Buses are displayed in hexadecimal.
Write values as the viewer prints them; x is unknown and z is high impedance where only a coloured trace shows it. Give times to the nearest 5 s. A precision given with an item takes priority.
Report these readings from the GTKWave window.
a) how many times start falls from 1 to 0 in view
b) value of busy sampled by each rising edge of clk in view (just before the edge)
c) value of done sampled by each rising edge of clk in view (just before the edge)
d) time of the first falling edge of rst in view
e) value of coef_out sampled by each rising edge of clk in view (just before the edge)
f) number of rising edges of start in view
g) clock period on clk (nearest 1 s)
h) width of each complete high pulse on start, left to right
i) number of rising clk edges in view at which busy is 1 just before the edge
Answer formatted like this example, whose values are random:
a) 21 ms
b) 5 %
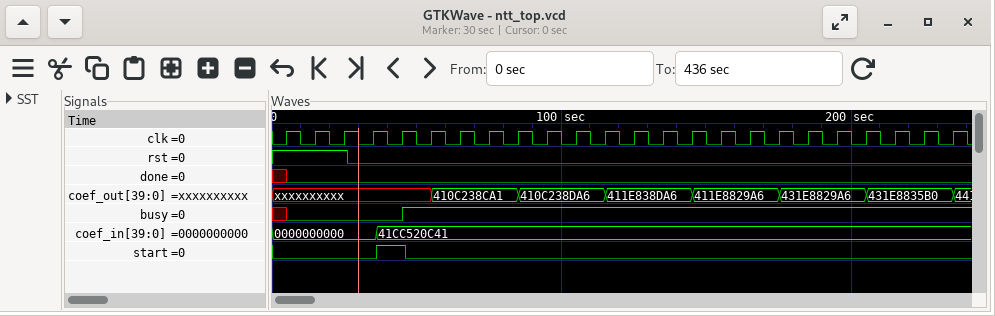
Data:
a) 1
b) x 0 0 0 0 1 1 1 1 1 1 1 1 1 1 1 1 1 1 1 1 1 1 1
c) x 0 0 0 0 0 0 0 0 0 0 0 0 0 0 0 0 0 0 0 0 0 0 0
d) 25 s
e) xxxxxxxxxx, xxxxxxxxxx, xxxxxxxxxx, xxxxxxxxxx, xxxxxxxxxx, xxxxxxxxxx, 410C238CA1, 410C238CA1, 410C238CA1, 410C238DA6, 410C238DA6, 410C238DA6, 411E838DA6, 411E838DA6, 411E838DA6, 411E8829A6, 411E8829A6, 411E8829A6, 431E8829A6, 431E8829A6, 431E8829A6, 431E8835B0, 431E8835B0, 431E8835B0
f) 1
g) 10 s
h) 10 s
i) 19
